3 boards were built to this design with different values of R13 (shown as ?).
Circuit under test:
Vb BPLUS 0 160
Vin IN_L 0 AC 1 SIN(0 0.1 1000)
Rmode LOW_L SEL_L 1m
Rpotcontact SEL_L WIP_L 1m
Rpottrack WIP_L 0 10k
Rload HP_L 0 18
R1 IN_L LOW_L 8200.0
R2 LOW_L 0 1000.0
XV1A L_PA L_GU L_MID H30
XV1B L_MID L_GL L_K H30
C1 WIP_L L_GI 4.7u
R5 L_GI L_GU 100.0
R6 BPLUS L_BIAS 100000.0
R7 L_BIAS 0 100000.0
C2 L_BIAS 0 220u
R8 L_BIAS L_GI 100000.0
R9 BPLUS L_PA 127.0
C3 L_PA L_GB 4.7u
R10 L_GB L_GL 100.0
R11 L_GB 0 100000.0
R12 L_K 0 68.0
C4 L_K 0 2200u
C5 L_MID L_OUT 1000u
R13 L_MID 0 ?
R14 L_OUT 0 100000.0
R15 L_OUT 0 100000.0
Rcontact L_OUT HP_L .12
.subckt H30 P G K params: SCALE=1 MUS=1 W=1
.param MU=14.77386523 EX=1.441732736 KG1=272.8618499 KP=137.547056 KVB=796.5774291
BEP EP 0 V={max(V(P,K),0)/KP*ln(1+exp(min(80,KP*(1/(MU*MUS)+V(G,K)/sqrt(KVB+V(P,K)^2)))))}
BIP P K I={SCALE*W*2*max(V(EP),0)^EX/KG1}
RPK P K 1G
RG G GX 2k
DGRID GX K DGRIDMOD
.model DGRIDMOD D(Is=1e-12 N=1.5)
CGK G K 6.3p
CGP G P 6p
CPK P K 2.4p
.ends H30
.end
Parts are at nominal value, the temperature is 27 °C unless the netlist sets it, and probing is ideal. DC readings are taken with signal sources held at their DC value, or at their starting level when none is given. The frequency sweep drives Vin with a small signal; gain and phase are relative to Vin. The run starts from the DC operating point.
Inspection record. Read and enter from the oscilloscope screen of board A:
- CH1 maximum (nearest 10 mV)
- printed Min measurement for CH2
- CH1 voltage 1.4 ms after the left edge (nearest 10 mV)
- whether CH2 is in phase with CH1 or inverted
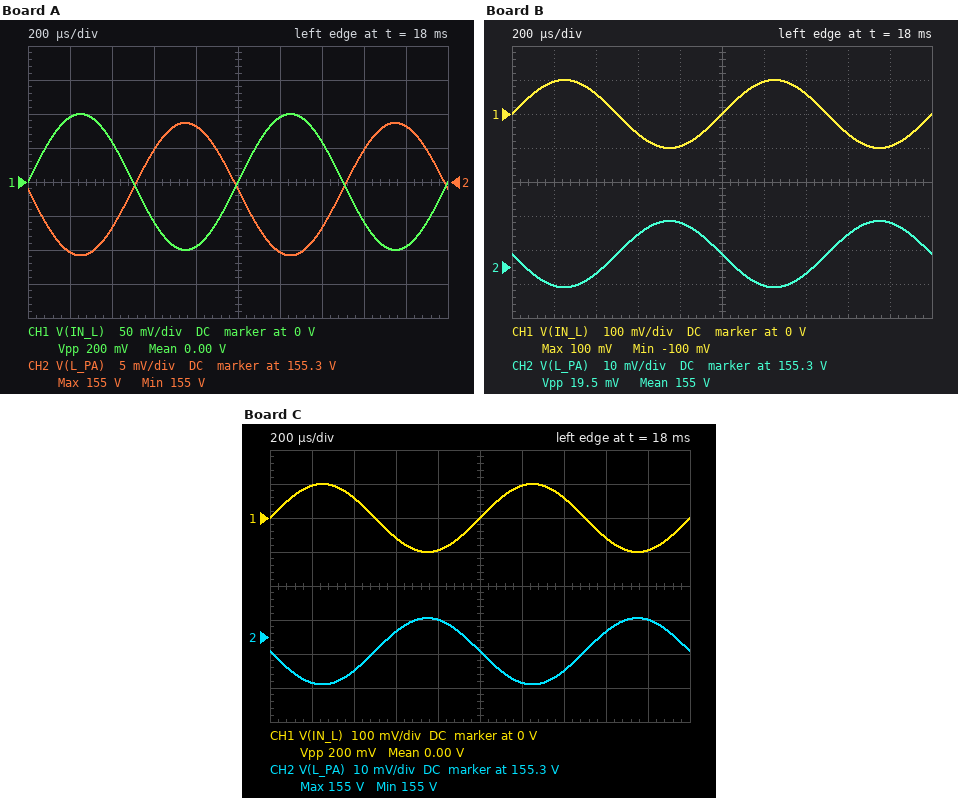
100 mV
155 V
60 mV
inverted
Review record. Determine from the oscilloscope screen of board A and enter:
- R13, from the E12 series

220 kΩ
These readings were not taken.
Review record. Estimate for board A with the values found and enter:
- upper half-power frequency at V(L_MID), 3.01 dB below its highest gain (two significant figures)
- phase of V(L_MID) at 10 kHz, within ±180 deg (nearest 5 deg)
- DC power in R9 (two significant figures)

7.2 Hz
0 deg
170 mW
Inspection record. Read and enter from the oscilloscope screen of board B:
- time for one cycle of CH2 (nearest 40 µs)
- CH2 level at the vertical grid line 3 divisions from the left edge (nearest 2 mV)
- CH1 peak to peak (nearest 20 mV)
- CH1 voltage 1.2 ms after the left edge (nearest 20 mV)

1.00 ms
155.310 V
200 mV
100 mV
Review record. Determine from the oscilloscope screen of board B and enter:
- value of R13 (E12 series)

180 kΩ
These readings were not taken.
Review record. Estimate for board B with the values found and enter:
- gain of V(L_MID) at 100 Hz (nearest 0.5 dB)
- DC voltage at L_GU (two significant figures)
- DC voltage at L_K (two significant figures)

-27.5 dB
80 V
2.5 V
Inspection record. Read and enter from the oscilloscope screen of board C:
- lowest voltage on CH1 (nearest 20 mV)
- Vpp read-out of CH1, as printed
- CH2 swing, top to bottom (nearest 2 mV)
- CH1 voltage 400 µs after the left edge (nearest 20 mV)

-100 mV
200 mV
20 mV
60 mV
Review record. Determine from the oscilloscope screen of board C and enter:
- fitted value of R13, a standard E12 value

120 kΩ
